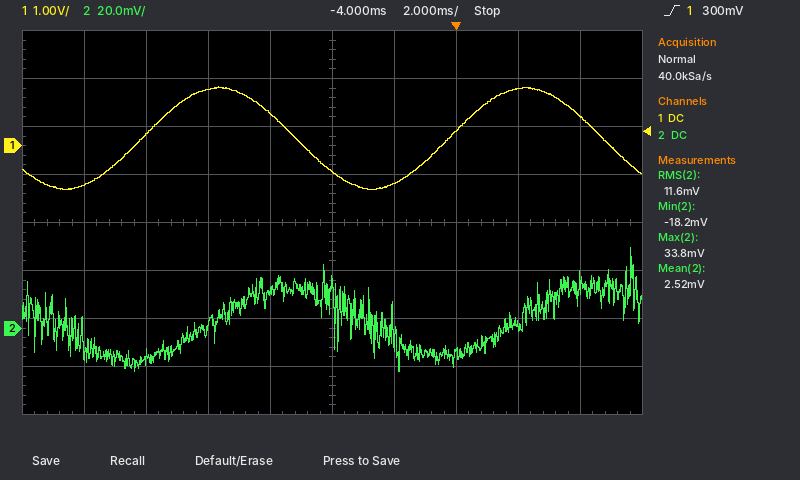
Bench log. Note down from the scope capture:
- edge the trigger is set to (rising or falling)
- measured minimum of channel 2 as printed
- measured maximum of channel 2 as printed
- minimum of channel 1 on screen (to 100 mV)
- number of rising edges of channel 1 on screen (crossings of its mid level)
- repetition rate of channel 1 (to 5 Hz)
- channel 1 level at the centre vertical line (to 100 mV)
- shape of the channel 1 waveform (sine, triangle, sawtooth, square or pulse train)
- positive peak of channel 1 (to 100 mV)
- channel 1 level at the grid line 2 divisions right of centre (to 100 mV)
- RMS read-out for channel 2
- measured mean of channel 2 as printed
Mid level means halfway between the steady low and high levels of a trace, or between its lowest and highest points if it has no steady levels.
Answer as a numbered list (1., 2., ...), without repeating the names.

1. rising
2. -18.2 mV
3. 33.8 mV
4. -900 mV
5. 2
6. 100 Hz
7. -500 mV
8. sine
9. 1.2 V
10. 300 mV
11. 11.6 mV
12. 2.52 mV
